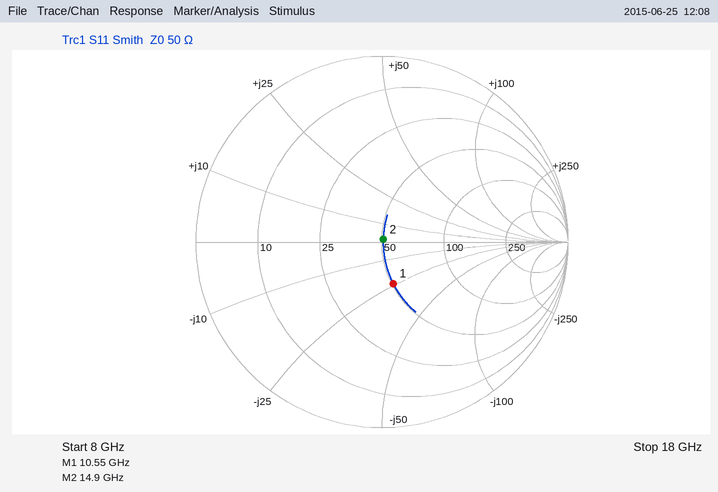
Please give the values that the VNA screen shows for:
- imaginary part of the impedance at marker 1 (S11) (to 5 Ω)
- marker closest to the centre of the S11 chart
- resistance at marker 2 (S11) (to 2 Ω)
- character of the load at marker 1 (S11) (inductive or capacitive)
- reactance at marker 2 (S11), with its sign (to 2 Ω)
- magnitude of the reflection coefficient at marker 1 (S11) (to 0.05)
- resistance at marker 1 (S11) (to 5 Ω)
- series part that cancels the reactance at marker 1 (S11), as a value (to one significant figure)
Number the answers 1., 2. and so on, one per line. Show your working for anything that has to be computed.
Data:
1. -25 Ω
2. marker 2
3. 50 Ω
4. capacitive
5. +2 Ω
6. 0.25
7. 50 Ω
8. L = 25 Ω/(2π × 10.55 GHz) ≈ 377 pH, so 400 pH to one significant figure
